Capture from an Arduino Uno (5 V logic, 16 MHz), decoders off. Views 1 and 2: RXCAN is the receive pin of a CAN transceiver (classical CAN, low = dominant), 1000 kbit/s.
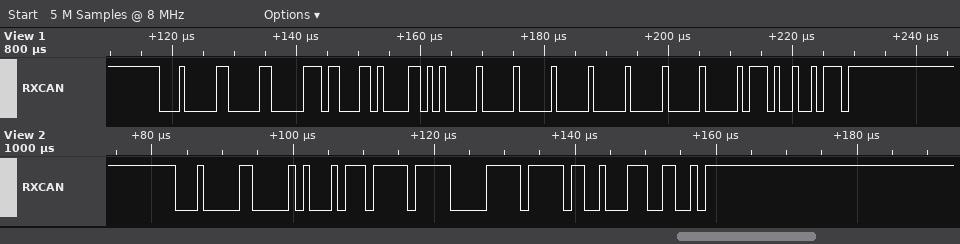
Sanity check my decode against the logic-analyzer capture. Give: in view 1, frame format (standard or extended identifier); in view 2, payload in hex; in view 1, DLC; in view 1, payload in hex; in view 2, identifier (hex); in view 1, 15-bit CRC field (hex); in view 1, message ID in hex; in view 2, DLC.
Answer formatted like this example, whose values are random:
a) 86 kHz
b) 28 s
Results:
a) standard
b) 5D FF 87 FF
c) 8
d) 36 34 35 00 00 00 00 00
e) 0x104
f) 0x3A4B
g) 0x104
h) 4
